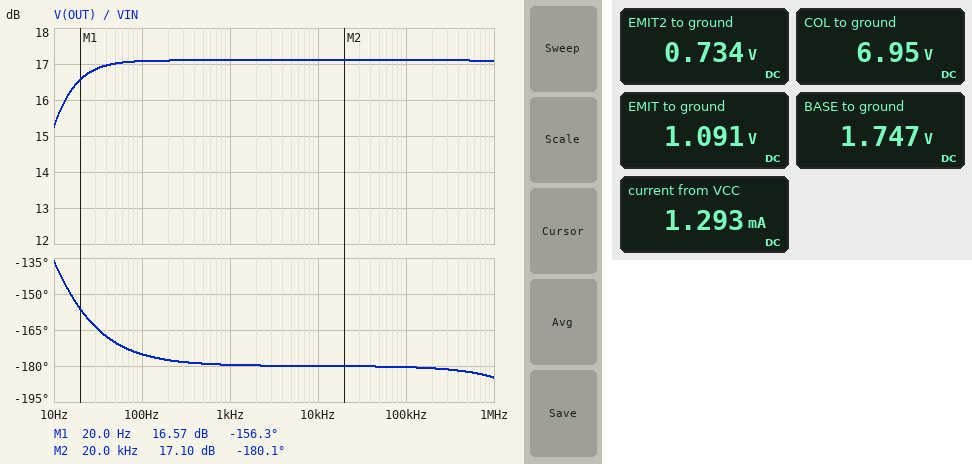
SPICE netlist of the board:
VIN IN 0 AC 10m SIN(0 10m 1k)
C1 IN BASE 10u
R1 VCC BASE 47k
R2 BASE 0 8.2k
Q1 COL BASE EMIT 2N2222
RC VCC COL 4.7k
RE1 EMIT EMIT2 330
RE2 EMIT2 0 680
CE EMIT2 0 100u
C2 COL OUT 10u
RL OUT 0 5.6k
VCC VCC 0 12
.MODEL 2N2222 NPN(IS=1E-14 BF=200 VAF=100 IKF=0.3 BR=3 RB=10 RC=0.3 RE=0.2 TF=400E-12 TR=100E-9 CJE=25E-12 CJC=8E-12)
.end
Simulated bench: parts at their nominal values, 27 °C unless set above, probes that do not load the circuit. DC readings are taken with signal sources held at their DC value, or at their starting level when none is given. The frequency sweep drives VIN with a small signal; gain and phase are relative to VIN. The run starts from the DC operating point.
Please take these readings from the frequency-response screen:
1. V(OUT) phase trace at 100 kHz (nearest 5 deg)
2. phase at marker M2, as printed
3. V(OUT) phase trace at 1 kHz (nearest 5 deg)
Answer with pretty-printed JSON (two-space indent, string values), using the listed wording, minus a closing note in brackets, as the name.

{
  "V(OUT) phase trace at 100 kHz": "-180 deg",
  "phase at marker M2, as printed": "-180.1 deg",
  "V(OUT) phase trace at 1 kHz": "-180 deg"
}
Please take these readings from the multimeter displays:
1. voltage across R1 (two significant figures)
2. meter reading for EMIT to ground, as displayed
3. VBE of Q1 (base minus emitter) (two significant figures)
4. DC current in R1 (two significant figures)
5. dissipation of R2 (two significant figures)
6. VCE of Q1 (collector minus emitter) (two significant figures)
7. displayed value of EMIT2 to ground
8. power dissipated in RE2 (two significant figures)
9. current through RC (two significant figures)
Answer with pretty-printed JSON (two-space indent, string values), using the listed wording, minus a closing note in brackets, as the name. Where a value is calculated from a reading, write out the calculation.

{
  "voltage across R1": "12 V - 1.747 V = 10 V",
  "meter reading for EMIT to ground, as displayed": "1.091 V",
  "VBE of Q1 (base minus emitter)": "1.747 V - 1.091 V = 660 mV",
  "DC current in R1": "(12 V - 1.747 V) / 47 kΩ = 220 µA",
  "dissipation of R2": "(1.747 V)^2 / 8.2 kΩ = 370 µW",
  "VCE of Q1 (collector minus emitter)": "6.95 V - 1.091 V = 5.9 V",
  "displayed value of EMIT2 to ground": "0.734 V",
  "power dissipated in RE2": "(734 mV)^2 / 680 Ω = 790 µW",
  "current through RC": "(12 V - 6.95 V) / 4.7 kΩ = 1.1 mA"
}
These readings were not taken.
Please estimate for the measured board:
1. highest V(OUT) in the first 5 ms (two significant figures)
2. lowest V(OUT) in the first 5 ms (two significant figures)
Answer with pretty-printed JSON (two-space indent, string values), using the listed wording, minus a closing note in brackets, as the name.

{
  "highest V(OUT) in the first 5 ms": "72 mV",
  "lowest V(OUT) in the first 5 ms": "-71 mV"
}
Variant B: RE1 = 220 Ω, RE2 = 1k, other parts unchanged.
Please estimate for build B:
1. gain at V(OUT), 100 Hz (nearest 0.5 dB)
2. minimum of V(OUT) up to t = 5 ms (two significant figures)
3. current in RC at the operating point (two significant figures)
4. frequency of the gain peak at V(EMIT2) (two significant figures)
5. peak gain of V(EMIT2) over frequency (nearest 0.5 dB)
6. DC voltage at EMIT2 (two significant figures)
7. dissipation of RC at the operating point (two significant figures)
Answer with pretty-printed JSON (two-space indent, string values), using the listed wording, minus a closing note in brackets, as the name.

{
  "gain at V(OUT), 100 Hz": "20.0 dB",
  "minimum of V(OUT) up to t = 5 ms": "-100 mV",
  "current in RC at the operating point": "900 µA",
  "frequency of the gain peak at V(EMIT2)": "4.3 Hz",
  "peak gain of V(EMIT2) over frequency": "-4.5 dB",
  "DC voltage at EMIT2": "900 mV",
  "dissipation of RC at the operating point": "3.8 mW"
}
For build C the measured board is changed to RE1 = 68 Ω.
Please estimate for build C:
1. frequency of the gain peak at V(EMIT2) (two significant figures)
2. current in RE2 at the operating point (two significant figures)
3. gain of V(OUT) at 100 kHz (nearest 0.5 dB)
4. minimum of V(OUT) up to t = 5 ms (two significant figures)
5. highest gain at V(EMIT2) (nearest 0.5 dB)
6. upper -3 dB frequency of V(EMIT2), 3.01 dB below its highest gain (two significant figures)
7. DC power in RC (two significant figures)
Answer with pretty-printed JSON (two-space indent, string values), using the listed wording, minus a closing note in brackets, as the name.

{
  "frequency of the gain peak at V(EMIT2)": "7.0 Hz",
  "current in RE2 at the operating point": "1.4 mA",
  "gain of V(OUT) at 100 kHz": "29.5 dB",
  "minimum of V(OUT) up to t = 5 ms": "-290 mV",
  "highest gain at V(EMIT2)": "-2.5 dB",
  "upper -3 dB frequency of V(EMIT2), 3.01 dB below its highest gain": "26 Hz",
  "DC power in RC": "9.5 mW"
}
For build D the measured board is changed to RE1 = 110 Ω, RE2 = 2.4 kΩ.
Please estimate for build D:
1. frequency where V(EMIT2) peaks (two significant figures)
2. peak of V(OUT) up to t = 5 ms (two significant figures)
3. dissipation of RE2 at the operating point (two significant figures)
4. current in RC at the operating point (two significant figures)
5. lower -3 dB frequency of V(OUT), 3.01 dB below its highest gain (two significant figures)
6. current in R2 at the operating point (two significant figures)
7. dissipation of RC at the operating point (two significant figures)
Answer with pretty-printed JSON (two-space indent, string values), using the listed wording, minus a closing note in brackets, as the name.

{
  "frequency where V(EMIT2) peaks": "4.8 Hz",
  "peak of V(OUT) up to t = 5 ms": "150 mV",
  "dissipation of RE2 at the operating point": "490 µW",
  "current in RC at the operating point": "450 µA",
  "lower -3 dB frequency of V(OUT), 3.01 dB below its highest gain": "11 Hz",
  "current in R2 at the operating point": "220 µA",
  "dissipation of RC at the operating point": "950 µW"
}
